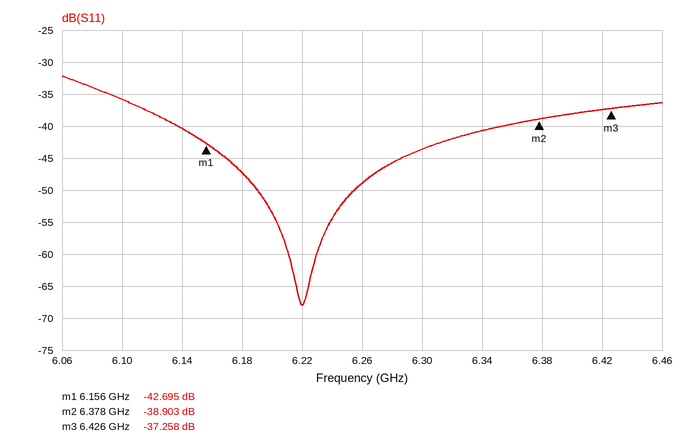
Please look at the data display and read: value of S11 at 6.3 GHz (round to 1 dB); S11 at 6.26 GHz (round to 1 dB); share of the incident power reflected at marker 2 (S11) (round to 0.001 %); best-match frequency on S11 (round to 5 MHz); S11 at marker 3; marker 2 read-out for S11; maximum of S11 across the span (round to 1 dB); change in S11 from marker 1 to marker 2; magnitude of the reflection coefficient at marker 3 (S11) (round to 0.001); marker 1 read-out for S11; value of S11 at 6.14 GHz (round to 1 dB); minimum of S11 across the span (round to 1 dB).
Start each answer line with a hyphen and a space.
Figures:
- -44 dB
- -49 dB
- 0.013 %
- 6.220 GHz
- -37.258 dB
- -38.903 dB
- -32 dB
- 3.792 dB
- 0.014
- -42.695 dB
- -40 dB
- -68 dB
